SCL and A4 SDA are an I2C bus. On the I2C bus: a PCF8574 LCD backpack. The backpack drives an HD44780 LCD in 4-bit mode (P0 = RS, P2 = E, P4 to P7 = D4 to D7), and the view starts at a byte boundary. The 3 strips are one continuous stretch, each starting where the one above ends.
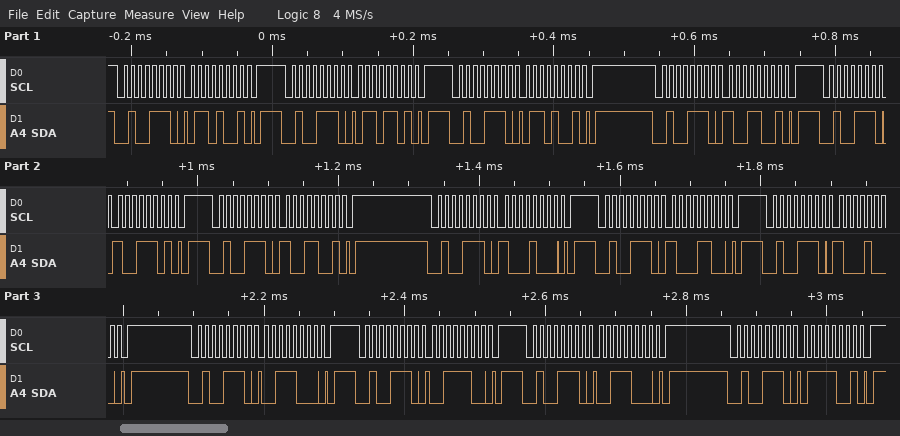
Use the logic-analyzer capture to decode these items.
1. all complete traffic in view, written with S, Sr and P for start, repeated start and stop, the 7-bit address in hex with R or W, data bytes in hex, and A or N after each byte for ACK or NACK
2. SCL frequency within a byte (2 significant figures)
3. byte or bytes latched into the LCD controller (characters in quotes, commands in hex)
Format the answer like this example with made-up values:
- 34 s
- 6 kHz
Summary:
- S 27W A 69 A P S 27W A 6D A P S 27W A 69 A P S 27W A 99 A P S 27W A 9D A P S 27W A 99 A P S 27W A 88 A P S 27W A 8C A P S 27W A 88 A P S 27W A 38 A P S 27W A 3C A P S 27W A 38 A P S 27W A 79 A P
- 100 kHz
- 'i' 0x83
